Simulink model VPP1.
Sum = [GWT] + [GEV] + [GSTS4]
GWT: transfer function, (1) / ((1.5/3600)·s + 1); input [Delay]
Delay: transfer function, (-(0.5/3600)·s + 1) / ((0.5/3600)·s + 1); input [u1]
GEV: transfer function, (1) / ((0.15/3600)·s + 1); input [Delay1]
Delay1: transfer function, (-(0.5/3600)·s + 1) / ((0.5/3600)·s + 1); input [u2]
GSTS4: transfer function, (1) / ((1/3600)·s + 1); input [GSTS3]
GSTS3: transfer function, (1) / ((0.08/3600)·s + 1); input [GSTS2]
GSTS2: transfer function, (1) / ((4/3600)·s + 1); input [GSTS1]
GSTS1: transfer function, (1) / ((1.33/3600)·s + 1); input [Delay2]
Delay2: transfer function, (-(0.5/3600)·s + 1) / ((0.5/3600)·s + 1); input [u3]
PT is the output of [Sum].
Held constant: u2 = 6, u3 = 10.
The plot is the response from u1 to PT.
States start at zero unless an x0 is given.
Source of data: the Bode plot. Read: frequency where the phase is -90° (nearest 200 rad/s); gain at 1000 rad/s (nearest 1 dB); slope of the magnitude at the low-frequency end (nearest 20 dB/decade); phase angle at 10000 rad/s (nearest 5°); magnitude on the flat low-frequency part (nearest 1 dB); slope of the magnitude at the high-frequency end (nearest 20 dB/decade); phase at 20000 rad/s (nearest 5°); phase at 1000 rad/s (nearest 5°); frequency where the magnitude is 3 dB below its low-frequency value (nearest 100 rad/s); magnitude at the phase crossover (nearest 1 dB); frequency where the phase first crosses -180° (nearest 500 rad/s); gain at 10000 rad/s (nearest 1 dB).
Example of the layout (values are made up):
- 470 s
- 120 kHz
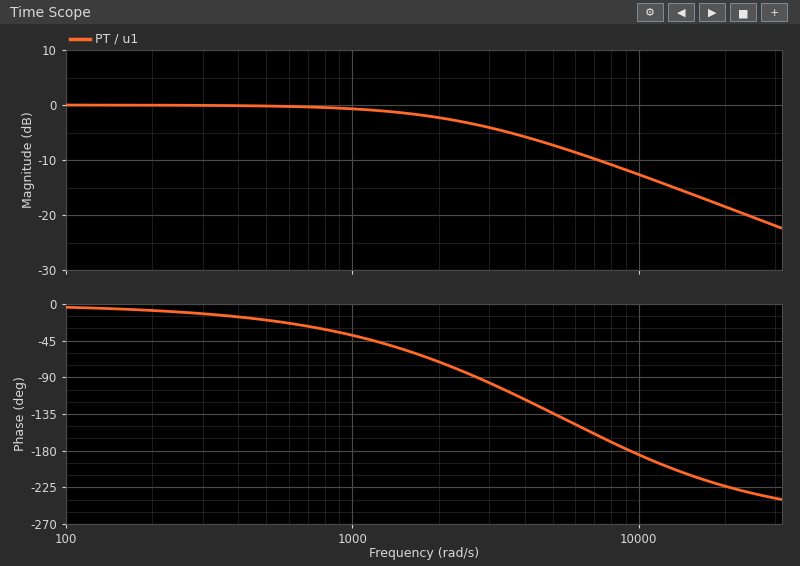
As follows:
- 2800 rad/s
- -1 dB
- 0 dB/decade
- -185°
- 0 dB
- -20 dB/decade
- -225°
- -40°
- 2400 rad/s
- -12 dB
- 9500 rad/s
- -13 dB
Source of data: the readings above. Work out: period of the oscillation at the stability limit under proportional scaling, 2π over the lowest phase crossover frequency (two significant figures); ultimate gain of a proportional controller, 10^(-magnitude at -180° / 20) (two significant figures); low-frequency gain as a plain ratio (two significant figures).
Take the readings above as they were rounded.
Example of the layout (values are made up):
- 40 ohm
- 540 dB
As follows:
- 0.00066 s
- 4.0
- 1.0
